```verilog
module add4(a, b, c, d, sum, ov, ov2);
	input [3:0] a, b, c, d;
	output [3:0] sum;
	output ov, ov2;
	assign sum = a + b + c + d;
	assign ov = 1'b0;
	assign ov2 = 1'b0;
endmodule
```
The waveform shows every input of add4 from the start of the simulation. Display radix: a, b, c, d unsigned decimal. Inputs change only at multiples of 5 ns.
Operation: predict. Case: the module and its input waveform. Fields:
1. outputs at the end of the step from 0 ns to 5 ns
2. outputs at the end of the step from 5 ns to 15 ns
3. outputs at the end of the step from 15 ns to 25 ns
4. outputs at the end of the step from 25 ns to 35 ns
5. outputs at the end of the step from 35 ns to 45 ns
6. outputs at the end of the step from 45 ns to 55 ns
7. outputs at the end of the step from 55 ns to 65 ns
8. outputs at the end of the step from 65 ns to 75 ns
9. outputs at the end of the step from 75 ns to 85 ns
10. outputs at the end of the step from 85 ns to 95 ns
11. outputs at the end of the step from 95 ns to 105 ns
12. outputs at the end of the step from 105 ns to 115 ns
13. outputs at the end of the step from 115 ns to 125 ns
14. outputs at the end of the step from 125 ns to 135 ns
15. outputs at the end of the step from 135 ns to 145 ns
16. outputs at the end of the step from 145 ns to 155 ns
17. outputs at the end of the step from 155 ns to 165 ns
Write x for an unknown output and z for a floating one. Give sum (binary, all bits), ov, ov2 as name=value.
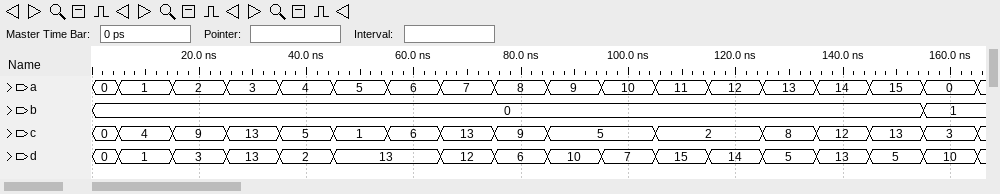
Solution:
sum=0000, ov=0, ov2=0
sum=0110, ov=0, ov2=0
sum=1110, ov=0, ov2=0
sum=1101, ov=0, ov2=0
sum=1011, ov=0, ov2=0
sum=0011, ov=0, ov2=0
sum=1001, ov=0, ov2=0
sum=0000, ov=0, ov2=0
sum=0111, ov=0, ov2=0
sum=1000, ov=0, ov2=0
sum=0110, ov=0, ov2=0
sum=1100, ov=0, ov2=0
sum=1100, ov=0, ov2=0
sum=1010, ov=0, ov2=0
sum=0111, ov=0, ov2=0
sum=0001, ov=0, ov2=0
sum=1110, ov=0, ov2=0
